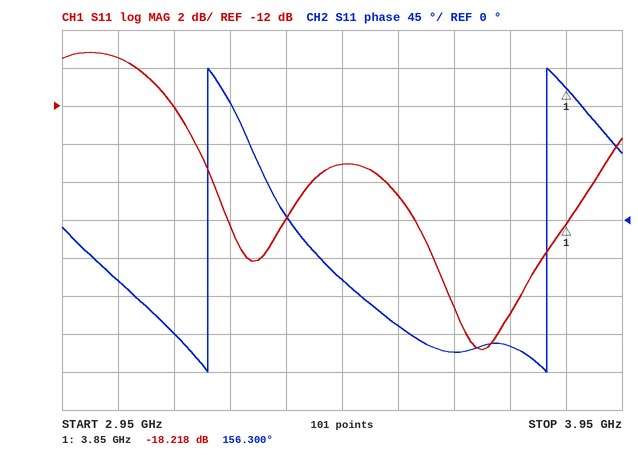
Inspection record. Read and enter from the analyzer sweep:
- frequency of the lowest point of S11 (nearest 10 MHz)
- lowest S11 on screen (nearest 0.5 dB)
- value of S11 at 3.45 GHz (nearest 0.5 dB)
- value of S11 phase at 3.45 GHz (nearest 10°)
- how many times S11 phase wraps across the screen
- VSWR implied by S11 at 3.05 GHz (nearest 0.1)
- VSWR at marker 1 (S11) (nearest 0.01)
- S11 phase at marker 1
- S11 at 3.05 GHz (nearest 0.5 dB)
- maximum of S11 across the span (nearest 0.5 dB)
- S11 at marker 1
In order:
3.70 GHz
-25.0 dB
-15.0 dB
-70°
2
2.0
1.28
156.300°
-9.5 dB
-9.0 dB
-18.218 dB
